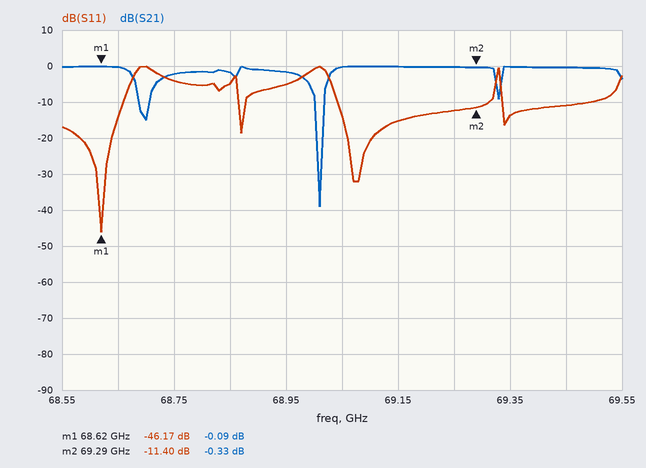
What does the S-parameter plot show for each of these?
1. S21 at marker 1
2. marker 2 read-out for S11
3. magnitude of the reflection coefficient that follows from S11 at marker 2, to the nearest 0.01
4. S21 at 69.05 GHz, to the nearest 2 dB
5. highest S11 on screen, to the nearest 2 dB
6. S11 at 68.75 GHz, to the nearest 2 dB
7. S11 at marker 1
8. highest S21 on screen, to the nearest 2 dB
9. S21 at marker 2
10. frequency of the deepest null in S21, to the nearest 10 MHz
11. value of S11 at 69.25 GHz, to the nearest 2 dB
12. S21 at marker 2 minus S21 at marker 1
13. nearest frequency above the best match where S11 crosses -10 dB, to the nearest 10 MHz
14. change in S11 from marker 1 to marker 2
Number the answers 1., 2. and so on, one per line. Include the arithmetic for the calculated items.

1. -0.09 dB
2. -11.40 dB
3. 10^(-11.4/20) ≈ 0.27
4. 0 dB
5. 0 dB
6. -4 dB
7. -46.17 dB
8. 0 dB
9. -0.33 dB
10. 69.01 GHz
11. -12 dB
12. -0.33 − (-0.09) = -0.24 dB
13. 68.66 GHz
14. -11.4 − (-46.17) = 34.77 dB
